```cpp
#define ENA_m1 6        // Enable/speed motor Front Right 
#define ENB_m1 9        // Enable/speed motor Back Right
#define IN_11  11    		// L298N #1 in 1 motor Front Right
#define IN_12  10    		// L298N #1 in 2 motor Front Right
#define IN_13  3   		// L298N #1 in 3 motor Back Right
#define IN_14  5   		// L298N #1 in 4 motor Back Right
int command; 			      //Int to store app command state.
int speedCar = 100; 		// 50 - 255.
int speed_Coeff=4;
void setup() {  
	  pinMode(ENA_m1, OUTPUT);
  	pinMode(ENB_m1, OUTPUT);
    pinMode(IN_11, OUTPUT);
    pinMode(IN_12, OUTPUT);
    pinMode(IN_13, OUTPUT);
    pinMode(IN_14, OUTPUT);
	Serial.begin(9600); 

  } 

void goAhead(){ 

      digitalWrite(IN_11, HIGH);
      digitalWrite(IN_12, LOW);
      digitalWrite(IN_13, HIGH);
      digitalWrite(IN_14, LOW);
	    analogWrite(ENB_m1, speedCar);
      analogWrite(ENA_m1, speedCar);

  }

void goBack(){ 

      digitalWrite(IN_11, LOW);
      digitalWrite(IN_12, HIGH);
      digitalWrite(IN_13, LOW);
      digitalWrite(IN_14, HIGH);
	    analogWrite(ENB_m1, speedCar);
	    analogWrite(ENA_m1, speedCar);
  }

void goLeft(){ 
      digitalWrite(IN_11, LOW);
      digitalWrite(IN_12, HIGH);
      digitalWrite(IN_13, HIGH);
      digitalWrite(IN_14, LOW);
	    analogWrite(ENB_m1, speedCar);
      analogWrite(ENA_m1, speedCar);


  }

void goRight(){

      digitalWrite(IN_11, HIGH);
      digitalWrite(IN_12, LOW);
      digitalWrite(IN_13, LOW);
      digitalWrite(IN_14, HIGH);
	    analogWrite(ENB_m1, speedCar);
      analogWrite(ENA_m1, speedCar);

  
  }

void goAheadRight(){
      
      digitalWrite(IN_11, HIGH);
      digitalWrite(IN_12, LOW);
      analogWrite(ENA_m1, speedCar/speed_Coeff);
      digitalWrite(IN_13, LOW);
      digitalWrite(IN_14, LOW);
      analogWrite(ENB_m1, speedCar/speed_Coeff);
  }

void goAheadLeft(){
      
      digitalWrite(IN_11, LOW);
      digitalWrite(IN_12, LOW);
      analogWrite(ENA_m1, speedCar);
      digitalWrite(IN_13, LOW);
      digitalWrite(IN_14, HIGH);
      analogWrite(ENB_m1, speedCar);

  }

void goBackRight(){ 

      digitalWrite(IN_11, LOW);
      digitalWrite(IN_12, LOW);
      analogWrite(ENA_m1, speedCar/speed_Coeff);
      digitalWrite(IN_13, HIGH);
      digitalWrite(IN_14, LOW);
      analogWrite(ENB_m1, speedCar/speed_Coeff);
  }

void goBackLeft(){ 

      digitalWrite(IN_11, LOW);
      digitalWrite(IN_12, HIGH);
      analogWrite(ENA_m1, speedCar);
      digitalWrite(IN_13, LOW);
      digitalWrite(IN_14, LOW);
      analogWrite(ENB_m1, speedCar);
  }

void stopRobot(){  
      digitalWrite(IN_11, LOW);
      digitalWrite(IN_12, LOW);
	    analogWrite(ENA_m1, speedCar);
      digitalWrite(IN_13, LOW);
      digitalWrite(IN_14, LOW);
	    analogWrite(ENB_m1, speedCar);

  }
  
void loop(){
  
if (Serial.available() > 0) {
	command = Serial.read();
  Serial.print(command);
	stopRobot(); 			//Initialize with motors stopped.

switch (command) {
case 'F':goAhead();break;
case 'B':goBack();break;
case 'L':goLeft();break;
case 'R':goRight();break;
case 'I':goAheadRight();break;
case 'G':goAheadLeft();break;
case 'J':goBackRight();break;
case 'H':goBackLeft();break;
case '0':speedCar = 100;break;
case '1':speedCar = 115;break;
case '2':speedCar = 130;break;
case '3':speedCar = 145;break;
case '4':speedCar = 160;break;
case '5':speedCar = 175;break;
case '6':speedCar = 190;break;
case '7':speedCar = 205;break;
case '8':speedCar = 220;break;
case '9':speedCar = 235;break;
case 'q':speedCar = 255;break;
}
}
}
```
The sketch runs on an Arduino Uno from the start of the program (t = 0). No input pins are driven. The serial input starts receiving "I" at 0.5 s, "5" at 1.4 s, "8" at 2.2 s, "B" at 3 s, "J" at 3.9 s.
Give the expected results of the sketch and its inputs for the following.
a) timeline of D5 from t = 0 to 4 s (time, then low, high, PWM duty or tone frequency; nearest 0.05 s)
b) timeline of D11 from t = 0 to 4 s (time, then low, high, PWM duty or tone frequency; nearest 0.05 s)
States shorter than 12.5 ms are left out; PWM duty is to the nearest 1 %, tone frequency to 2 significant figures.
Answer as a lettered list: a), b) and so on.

a) 0 s low; 3 s high; 3.9 s low
b) 0 s low; 0.5 s high; 1.4 s low
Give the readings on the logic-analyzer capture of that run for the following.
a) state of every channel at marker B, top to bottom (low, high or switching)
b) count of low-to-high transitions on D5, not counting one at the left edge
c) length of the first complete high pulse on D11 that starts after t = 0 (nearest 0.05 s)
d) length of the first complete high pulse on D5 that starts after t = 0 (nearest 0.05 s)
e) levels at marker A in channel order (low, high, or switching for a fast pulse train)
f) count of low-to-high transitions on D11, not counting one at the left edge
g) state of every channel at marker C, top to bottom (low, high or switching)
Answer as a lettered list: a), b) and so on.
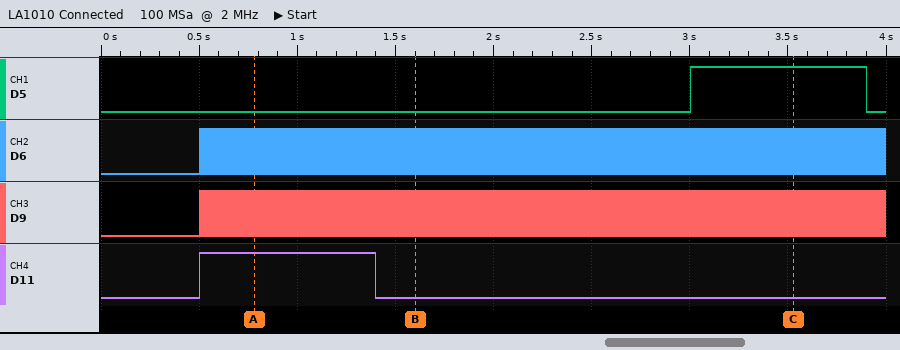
a) D5 low, D6 switching, D9 switching, D11 low
b) 1
c) 0.90 s
d) 0.90 s
e) D5 low, D6 switching, D9 switching, D11 high
f) 1
g) D5 high, D6 switching, D9 switching, D11 low
